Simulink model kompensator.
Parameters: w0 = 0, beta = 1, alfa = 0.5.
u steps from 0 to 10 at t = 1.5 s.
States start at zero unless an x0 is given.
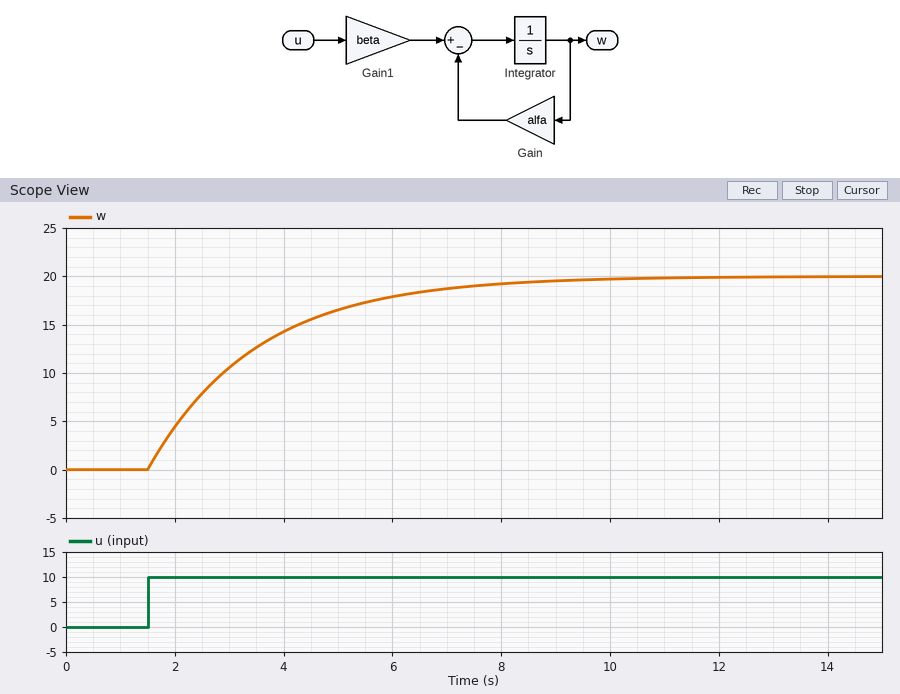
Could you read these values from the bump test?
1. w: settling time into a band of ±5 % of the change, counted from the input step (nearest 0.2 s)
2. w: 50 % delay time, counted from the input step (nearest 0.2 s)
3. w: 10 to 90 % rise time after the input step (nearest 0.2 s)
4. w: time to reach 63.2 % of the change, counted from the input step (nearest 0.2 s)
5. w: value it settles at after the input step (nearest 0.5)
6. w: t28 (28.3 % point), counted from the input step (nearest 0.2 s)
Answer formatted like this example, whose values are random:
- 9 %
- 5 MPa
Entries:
- 6.0 s
- 1.4 s
- 4.4 s
- 2.0 s
- 20.0
- 0.6 s
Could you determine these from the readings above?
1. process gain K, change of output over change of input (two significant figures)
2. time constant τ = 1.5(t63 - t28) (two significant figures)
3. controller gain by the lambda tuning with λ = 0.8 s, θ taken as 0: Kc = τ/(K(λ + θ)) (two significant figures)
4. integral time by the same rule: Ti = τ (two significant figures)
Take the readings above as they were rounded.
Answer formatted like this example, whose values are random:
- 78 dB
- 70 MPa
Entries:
- 2.0
- 2.1 s
- 1.3
- 2.1 s
